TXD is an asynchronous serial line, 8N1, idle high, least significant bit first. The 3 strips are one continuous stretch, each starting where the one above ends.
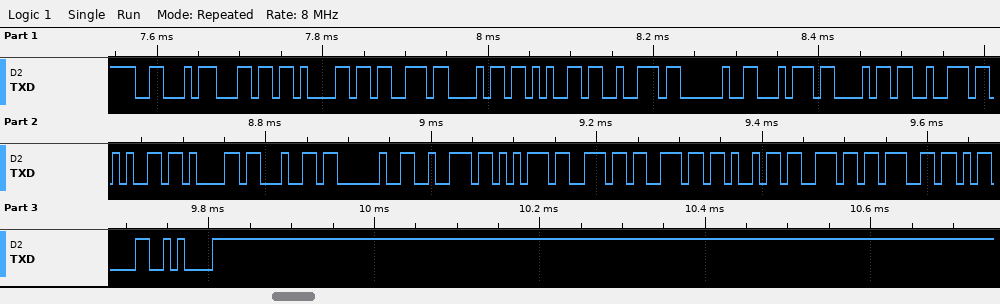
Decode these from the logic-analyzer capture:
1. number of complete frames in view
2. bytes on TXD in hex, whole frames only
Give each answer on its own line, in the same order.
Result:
24
46 6C 61 73 68 65 72 20 74 68 72 65 61 64 20 72 75 6E 6E 69 6E 67 0D 0A
